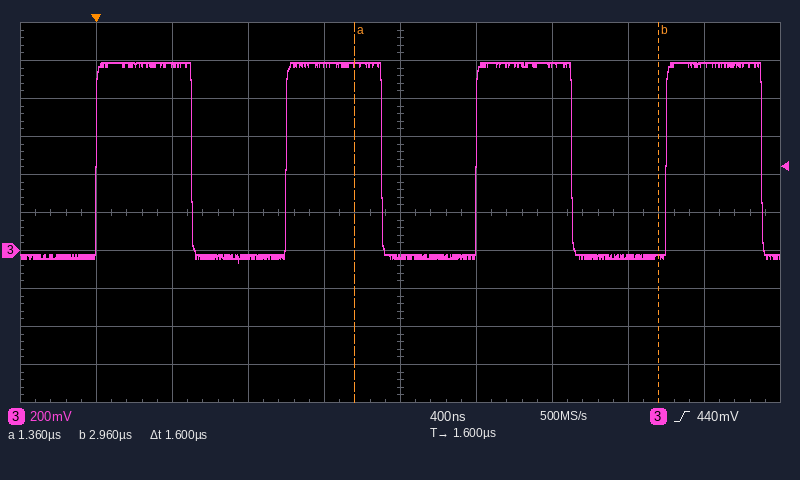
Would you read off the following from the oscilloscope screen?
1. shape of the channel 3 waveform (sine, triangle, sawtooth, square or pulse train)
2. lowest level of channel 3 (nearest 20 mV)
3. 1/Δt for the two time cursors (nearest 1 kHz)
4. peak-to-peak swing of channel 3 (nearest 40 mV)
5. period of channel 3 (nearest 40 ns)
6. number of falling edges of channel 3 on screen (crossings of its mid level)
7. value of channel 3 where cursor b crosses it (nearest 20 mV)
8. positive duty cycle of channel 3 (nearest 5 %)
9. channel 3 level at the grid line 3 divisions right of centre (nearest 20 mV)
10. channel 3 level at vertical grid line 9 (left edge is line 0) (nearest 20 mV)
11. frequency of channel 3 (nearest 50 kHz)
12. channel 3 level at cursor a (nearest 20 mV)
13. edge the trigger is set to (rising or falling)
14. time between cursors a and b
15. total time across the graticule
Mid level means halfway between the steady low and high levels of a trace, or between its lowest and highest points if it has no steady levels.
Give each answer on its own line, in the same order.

square
-60 mV
625 kHz
1.04 V
1.00 µs
4
-40 mV
50 %
-40 mV
980 mV
1.00 MHz
980 mV
rising
1.6 µs
4 µs
